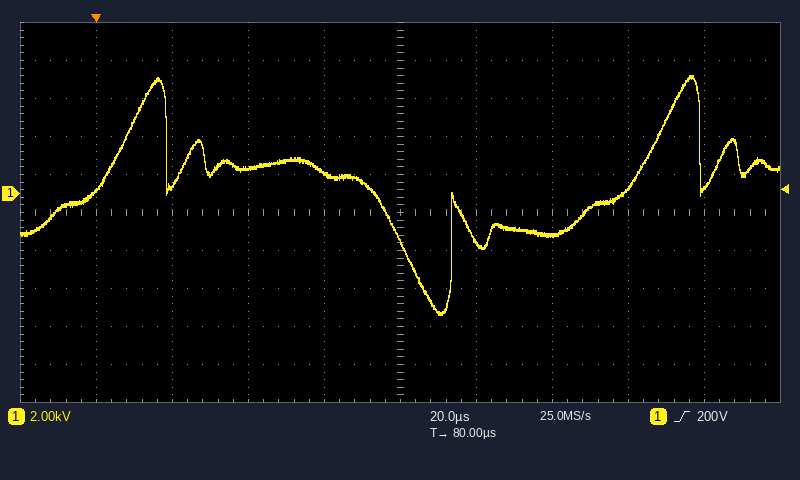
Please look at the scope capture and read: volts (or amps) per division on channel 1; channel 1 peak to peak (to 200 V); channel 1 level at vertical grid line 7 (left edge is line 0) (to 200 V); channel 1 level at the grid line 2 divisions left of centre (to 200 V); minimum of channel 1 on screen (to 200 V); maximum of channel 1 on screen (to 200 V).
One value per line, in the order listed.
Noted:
2 kV
12.6 kV
-2.2 kV
1.4 kV
-6.4 kV
6.2 kV
